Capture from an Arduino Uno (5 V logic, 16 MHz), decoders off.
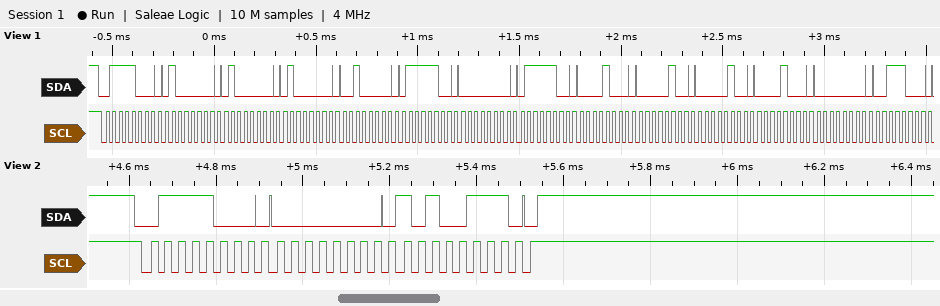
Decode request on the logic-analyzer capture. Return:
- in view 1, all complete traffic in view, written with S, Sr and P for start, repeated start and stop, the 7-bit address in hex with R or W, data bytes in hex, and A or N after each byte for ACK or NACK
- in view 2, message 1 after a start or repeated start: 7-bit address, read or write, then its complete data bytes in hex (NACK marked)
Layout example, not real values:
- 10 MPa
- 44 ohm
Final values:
- S 3CW A 40 A 40 A 40 A 20 A 7C A 00 A 7C A 08 A 04 A 04 A 08 A 00 A 38 A
- 0x3C write: 00 A7
